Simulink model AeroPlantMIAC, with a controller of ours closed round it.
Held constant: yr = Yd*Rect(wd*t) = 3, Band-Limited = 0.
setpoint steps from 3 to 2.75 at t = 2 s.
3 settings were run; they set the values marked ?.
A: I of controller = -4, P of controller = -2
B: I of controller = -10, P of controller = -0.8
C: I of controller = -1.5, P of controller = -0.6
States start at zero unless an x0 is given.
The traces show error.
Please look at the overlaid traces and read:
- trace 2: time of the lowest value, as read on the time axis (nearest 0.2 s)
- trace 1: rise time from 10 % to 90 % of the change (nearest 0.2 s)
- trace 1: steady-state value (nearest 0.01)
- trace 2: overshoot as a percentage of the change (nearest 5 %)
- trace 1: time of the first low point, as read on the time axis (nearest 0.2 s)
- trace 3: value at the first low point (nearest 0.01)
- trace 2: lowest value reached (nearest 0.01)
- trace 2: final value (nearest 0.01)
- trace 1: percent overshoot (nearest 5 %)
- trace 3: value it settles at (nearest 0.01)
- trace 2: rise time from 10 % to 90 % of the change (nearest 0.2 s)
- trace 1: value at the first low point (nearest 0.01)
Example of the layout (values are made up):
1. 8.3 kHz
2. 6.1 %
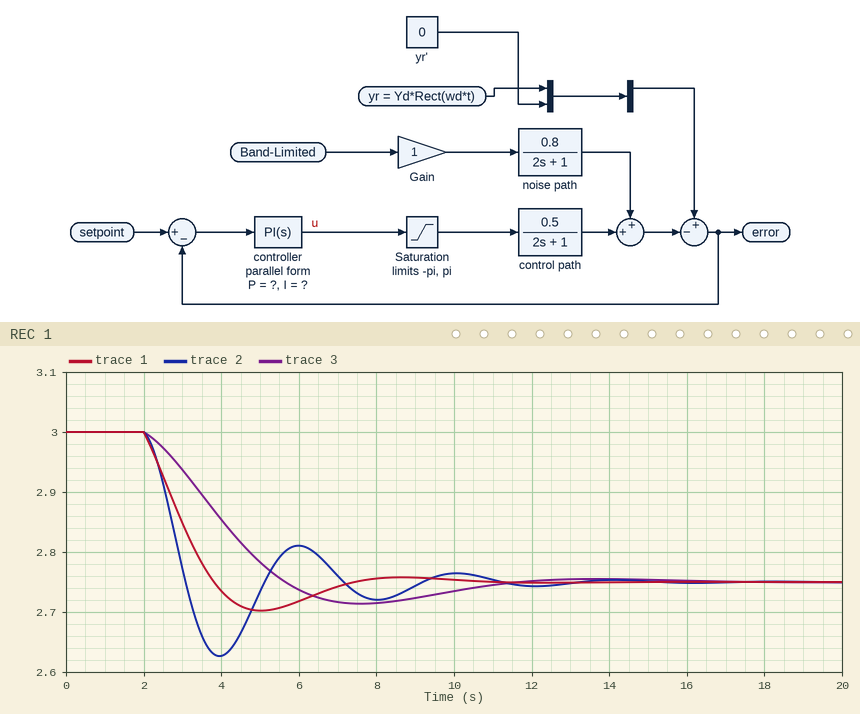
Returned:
1. 4.0 s
2. 1.4 s
3. 2.75
4. 50 %
5. 5.0 s
6. 2.71
7. 2.63
8. 2.75
9. 20 %
10. 2.75
11. 0.8 s
12. 2.70
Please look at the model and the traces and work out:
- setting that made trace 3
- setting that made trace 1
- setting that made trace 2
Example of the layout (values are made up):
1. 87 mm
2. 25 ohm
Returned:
1. C
2. A
3. B
